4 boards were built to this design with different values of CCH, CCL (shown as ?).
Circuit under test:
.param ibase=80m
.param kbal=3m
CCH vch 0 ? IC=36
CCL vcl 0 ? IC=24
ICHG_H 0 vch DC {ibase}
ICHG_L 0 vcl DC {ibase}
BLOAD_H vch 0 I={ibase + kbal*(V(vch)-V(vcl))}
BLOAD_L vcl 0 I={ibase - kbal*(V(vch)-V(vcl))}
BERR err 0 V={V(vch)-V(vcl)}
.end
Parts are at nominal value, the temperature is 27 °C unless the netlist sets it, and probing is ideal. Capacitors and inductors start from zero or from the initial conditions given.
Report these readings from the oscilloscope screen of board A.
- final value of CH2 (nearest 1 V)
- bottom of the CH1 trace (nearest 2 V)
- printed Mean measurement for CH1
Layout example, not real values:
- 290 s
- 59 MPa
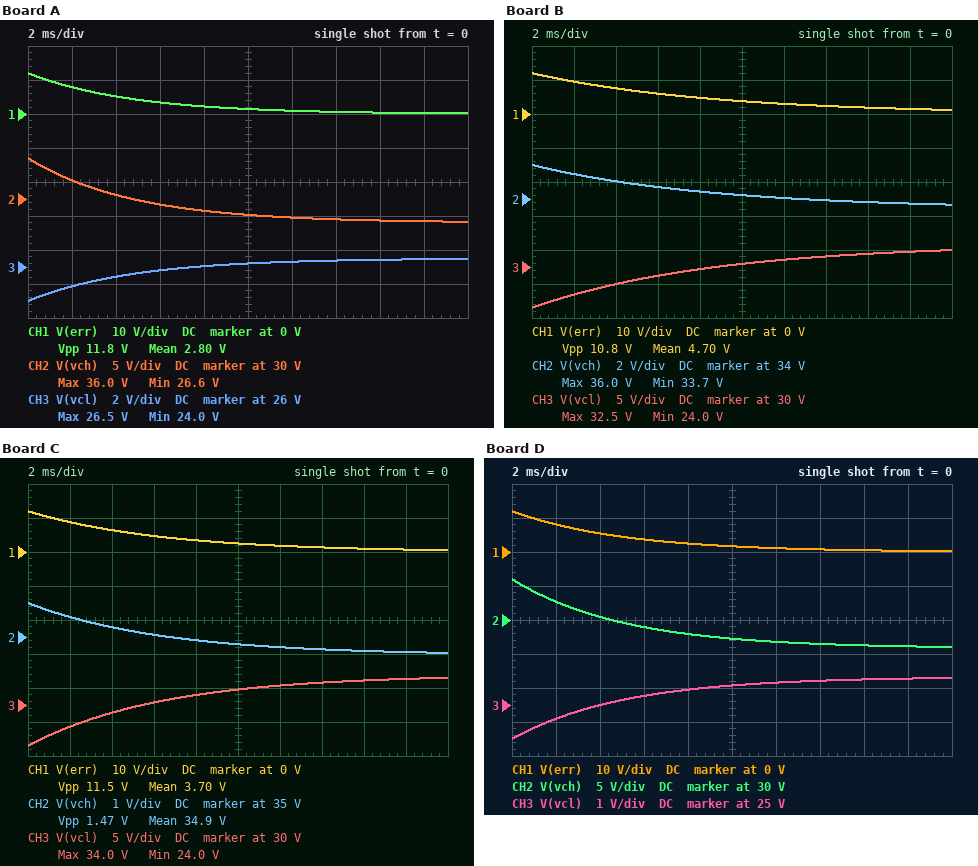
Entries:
- 27 V
- 0 V
- 2.80 V
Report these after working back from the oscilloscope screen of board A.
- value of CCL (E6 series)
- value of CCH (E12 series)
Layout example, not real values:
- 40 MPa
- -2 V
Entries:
- 68 µF
- 18 µF
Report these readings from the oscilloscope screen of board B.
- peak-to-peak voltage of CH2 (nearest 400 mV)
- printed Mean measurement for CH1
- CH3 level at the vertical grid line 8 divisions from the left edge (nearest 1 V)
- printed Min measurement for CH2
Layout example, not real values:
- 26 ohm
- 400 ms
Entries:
- 2.4 V
- 4.70 V
- 32 V
- 33.7 V
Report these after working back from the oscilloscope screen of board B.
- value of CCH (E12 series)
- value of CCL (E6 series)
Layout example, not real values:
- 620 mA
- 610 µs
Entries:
- 120 µF
- 33 µF
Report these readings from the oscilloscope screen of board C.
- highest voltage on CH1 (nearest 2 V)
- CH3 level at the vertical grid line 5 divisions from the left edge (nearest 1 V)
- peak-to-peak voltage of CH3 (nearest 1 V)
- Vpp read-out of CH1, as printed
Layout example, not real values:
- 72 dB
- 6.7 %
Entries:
- 12 V
- 32 V
- 10 V
- 11.5 V
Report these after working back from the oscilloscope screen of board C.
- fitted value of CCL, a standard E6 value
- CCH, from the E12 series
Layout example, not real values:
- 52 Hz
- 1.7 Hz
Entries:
- 22 µF
- 150 µF
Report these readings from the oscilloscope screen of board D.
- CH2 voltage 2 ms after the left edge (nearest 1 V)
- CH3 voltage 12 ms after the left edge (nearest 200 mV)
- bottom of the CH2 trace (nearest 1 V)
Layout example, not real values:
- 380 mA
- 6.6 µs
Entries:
- 33 V
- 25.6 V
- 26 V
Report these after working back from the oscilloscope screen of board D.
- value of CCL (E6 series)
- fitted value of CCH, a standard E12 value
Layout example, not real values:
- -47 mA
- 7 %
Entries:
- 100 µF
- 18 µF
